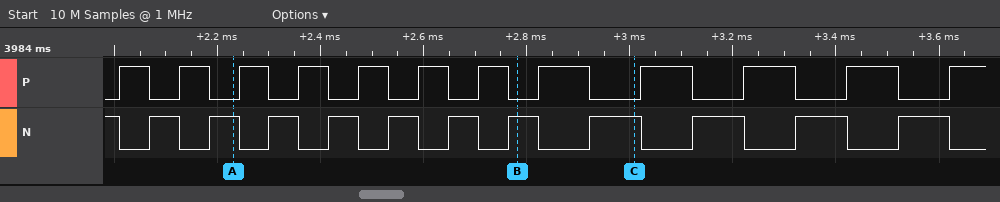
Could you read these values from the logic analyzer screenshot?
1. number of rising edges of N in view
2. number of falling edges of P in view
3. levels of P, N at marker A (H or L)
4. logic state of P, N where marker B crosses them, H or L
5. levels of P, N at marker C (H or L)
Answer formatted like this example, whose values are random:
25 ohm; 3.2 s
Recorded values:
11; 11; P=L, N=H; P=L, N=H; P=L, N=H
